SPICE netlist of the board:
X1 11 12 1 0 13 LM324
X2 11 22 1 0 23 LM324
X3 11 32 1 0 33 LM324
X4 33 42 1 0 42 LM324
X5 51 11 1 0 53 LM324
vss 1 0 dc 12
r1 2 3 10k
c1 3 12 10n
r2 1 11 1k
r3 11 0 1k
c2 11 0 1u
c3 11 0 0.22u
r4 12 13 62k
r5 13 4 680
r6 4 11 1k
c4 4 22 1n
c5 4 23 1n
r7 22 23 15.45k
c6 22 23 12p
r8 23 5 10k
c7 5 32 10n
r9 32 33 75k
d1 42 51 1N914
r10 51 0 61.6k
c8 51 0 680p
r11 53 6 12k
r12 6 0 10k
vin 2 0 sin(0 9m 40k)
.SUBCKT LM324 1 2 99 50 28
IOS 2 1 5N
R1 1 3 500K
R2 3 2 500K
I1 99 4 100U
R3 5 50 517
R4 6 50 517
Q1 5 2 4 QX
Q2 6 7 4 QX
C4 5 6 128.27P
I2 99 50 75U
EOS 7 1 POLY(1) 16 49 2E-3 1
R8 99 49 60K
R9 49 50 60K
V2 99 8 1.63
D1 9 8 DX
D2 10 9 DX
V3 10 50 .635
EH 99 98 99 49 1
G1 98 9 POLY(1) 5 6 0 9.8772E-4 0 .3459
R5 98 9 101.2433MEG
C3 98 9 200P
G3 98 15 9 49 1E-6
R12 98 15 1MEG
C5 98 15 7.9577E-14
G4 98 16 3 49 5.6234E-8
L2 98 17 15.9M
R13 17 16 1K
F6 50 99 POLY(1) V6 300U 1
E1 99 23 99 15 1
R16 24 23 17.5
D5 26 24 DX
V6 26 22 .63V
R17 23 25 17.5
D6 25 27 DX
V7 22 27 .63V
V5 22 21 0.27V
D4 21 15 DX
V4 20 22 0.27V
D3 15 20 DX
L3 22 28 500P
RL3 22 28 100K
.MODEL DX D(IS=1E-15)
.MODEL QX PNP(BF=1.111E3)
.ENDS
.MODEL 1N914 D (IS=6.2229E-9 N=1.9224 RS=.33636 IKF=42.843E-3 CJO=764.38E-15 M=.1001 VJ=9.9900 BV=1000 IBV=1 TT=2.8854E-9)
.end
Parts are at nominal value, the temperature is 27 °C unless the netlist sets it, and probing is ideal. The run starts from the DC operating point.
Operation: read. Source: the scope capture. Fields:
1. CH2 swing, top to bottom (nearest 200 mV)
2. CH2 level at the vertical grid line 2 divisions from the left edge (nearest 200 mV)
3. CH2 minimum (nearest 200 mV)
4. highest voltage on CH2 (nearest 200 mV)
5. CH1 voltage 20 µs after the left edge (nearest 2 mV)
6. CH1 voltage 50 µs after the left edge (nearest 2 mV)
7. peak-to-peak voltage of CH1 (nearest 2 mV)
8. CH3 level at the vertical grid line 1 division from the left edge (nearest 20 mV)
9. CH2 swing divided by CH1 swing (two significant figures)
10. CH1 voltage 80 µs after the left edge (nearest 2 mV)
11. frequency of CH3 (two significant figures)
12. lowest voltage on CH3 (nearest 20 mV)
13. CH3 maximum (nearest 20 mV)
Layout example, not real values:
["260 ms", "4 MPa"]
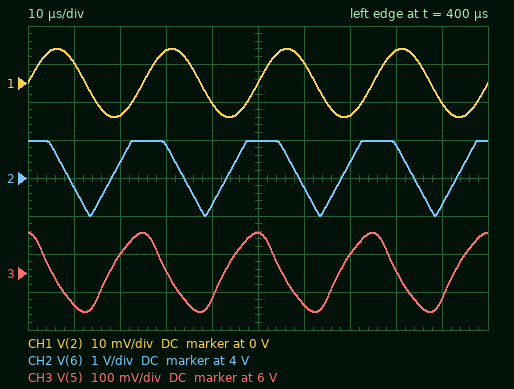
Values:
["2.0 V", "4.4 V", "3.0 V", "5.0 V", "-8 mV", "0 V", "18 mV", "5.92 V", "110", "8 mV", "40 kHz", "5.90 V", "6.10 V"]
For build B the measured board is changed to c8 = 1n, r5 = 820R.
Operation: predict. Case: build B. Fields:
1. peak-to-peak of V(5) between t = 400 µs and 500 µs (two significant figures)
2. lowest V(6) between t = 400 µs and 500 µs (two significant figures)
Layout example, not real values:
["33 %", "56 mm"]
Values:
["200 mV", "3.9 V"]
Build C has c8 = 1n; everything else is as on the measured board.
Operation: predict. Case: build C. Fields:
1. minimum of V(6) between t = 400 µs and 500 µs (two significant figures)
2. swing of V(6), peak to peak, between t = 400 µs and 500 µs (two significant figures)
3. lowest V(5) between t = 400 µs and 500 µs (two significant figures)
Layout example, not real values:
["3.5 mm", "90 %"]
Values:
["4.0 V", "960 mV", "5.9 V"]
